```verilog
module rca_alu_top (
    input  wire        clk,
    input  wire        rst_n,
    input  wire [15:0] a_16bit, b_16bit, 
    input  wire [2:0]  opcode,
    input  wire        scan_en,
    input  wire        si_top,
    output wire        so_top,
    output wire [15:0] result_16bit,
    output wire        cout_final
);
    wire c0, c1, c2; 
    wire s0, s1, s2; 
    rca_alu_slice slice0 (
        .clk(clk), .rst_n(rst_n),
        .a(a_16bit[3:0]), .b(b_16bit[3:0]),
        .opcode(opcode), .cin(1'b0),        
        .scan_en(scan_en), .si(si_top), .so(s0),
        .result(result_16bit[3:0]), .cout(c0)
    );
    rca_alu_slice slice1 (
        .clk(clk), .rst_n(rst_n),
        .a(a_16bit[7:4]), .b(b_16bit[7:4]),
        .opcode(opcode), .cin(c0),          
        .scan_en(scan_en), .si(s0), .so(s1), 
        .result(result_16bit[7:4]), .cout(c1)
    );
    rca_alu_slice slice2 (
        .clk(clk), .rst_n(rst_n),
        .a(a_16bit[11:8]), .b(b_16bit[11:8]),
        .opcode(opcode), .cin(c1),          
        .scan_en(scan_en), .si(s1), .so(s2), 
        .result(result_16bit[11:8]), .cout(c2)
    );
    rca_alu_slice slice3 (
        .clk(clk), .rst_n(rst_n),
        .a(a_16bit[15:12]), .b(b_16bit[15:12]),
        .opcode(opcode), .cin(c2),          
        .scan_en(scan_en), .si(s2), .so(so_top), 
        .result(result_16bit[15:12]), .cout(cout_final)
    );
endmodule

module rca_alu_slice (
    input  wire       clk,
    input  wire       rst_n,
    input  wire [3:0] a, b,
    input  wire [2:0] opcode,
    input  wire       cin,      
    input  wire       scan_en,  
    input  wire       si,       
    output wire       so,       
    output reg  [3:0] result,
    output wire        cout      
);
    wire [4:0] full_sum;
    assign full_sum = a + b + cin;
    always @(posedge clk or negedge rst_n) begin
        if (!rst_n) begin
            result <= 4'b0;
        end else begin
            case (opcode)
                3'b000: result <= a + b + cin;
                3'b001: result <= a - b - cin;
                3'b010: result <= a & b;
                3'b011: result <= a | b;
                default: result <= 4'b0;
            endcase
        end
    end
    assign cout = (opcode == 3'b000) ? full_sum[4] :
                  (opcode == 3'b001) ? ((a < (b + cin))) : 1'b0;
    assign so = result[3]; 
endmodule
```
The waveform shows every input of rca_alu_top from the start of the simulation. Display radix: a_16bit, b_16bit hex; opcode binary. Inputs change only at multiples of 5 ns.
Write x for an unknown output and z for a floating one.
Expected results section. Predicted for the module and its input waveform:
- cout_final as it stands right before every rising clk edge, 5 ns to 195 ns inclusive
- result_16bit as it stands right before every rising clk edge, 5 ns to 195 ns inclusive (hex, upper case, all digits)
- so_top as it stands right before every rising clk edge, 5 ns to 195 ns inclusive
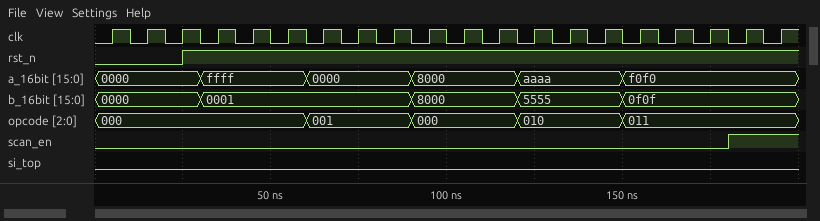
0 0 0 1 1 1 1 1 1 1 1 1 0 0 0 0 0 0 0 0
0000, 0000, 0000, 0000, 0000, 0000, 0000, FFFF, FFFF, FFFF, 0000, 0000, 0000, 0000, 0000, 0000, FFFF, FFFF, FFFF, FFFF
0 0 0 0 0 0 0 1 1 1 0 0 0 0 0 0 1 1 1 1
